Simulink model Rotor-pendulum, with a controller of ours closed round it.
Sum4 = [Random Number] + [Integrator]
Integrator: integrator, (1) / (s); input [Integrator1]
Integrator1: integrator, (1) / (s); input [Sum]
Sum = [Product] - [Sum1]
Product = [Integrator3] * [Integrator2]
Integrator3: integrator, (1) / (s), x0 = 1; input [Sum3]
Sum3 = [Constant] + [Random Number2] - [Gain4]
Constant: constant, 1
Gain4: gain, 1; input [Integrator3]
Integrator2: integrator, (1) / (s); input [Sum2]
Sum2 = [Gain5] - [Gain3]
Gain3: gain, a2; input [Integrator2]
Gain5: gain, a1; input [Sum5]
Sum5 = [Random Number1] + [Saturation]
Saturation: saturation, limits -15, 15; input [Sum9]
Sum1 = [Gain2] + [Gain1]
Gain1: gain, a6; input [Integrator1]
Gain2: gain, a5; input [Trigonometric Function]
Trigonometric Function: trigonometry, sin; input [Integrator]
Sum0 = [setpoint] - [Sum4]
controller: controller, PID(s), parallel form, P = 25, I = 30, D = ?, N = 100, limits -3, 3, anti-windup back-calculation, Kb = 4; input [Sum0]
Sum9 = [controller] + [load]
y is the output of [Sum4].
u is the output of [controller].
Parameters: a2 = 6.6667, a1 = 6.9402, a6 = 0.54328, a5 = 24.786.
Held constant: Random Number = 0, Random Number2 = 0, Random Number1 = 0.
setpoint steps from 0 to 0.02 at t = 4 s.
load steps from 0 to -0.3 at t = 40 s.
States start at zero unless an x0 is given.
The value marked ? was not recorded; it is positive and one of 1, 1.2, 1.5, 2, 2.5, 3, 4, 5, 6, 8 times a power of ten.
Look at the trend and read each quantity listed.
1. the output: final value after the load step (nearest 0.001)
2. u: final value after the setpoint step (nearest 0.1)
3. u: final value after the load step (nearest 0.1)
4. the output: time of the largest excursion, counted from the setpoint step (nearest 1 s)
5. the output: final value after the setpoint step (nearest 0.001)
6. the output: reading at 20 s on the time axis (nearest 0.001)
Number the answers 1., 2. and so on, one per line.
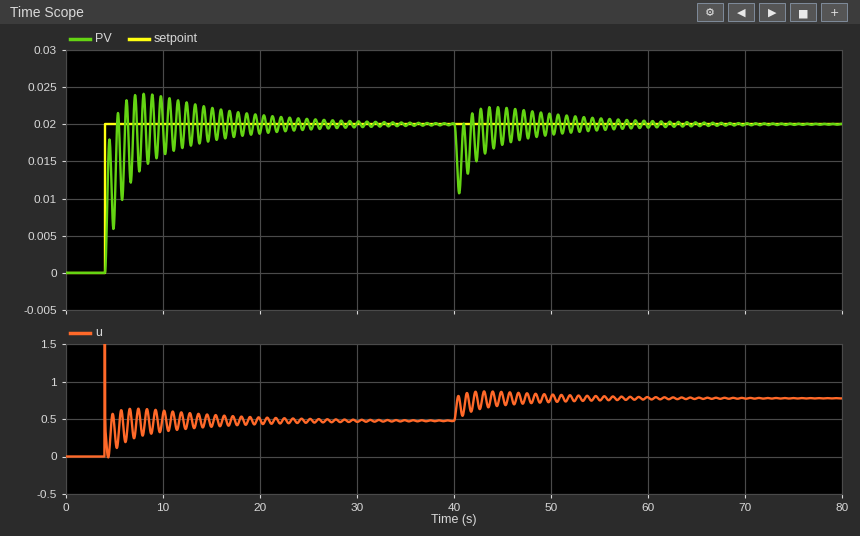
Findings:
1. 0.020
2. 0.5
3. 0.8
4. 4 s
5. 0.020
6. 0.019
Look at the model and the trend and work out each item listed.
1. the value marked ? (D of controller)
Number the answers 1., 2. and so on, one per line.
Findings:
1. 4
